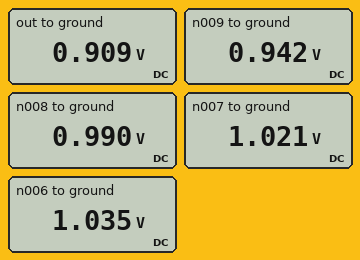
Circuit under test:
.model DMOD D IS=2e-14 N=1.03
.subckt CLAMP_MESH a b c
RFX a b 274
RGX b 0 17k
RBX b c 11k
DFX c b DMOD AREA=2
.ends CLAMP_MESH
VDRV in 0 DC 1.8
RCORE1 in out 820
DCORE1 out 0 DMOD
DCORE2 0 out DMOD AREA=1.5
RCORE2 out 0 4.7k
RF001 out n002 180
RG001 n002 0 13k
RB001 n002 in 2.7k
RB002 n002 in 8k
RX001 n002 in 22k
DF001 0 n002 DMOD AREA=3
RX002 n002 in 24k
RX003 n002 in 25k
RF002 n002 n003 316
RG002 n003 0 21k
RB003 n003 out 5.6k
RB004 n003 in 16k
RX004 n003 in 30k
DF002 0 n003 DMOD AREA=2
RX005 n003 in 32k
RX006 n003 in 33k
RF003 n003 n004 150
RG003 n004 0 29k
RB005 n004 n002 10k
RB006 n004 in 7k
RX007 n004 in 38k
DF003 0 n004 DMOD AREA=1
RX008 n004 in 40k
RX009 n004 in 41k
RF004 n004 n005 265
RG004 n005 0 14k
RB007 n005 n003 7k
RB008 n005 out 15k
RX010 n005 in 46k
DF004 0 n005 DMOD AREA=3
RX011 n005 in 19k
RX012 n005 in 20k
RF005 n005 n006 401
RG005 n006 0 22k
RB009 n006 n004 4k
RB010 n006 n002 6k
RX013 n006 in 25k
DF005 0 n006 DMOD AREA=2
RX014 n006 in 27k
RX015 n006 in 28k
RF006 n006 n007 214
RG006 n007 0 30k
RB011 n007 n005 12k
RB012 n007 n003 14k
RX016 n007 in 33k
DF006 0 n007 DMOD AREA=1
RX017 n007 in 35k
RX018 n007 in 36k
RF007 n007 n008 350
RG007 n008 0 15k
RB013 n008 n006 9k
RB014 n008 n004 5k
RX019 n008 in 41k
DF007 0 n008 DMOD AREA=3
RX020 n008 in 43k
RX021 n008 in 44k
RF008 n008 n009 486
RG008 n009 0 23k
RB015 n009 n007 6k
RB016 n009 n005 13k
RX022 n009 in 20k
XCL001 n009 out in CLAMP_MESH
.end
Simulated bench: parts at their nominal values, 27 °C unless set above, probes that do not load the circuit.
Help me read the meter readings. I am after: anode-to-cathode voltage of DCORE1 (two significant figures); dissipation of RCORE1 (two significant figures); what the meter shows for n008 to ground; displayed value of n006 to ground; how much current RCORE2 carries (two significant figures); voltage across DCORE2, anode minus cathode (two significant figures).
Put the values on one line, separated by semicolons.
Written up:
910 mV; 970 µW; 0.990 V; 1.035 V; 190 µA; -910 mV
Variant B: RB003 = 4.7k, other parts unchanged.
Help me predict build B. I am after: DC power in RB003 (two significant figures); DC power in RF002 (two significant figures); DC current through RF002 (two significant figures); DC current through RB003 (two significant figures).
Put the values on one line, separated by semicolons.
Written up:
3.8 µW; 4.1 µW; 110 µA; 28 µA
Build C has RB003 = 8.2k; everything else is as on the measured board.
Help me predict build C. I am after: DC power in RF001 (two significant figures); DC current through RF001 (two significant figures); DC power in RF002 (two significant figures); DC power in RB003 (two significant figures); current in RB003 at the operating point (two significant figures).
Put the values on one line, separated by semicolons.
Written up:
54 µW; 550 µA; 4.7 µW; 2.3 µW; 17 µA
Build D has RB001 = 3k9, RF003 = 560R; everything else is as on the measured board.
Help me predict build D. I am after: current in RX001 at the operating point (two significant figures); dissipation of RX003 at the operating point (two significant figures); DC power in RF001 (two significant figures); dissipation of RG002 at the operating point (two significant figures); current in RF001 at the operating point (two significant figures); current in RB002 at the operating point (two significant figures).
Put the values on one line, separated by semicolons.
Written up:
37 µA; 26 µW; 38 µW; 50 µW; 460 µA; 100 µA
